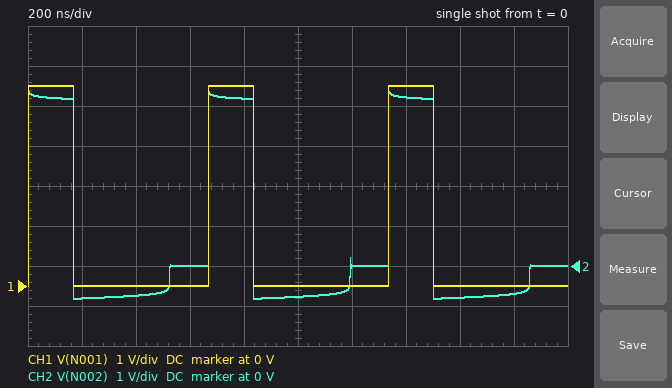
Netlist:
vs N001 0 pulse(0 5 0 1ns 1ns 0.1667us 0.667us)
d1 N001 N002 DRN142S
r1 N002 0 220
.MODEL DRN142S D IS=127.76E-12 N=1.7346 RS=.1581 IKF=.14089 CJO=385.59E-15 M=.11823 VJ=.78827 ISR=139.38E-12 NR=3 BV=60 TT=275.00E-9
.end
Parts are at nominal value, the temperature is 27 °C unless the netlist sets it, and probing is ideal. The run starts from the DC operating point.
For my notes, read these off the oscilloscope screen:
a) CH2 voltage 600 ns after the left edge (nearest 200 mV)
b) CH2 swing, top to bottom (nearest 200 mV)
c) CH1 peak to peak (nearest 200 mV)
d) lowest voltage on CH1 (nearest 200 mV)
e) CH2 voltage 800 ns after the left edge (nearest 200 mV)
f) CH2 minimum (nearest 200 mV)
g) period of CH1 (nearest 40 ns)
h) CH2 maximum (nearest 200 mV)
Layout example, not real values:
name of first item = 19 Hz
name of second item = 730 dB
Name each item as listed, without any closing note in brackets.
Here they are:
CH2 voltage 600 ns after the left edge = 0 V
CH2 swing, top to bottom = 5.2 V
CH1 peak to peak = 5.0 V
lowest voltage on CH1 = 0 V
CH2 voltage 800 ns after the left edge = 4.2 V
CH2 minimum = -800 mV
period of CH1 = 680 ns
CH2 maximum = 4.4 V
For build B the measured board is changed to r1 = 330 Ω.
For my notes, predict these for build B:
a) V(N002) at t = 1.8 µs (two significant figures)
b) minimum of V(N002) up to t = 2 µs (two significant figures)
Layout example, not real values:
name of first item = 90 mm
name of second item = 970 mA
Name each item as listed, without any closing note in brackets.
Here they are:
V(N002) at t = 1.8 µs = -680 mV
minimum of V(N002) up to t = 2 µs = -800 mV
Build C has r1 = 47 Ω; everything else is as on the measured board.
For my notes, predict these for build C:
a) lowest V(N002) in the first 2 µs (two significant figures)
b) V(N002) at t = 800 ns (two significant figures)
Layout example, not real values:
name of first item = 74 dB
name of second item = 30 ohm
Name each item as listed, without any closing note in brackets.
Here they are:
lowest V(N002) in the first 2 µs = -900 mV
V(N002) at t = 800 ns = 4.1 V
